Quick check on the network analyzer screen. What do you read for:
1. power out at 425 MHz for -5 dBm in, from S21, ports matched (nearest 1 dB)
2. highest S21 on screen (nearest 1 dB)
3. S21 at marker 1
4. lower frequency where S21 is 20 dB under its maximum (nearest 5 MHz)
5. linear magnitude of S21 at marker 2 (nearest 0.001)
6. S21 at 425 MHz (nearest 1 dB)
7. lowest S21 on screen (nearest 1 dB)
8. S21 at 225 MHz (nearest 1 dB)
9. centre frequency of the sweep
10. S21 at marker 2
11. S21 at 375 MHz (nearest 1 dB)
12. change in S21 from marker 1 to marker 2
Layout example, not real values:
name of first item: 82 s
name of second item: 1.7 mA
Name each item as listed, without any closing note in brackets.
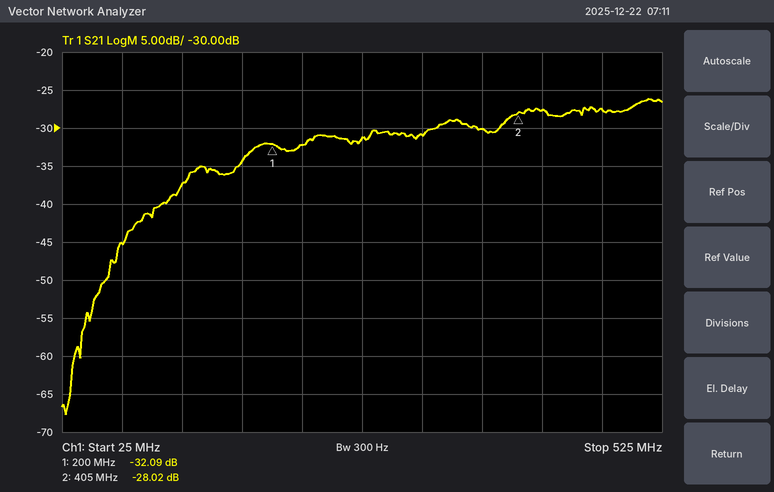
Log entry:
power out at 425 MHz for -5 dBm in, from S21, ports matched: -33 dBm
highest S21 on screen: -26 dB
S21 at marker 1: -32.09 dB
lower frequency where S21 is 20 dB under its maximum: 70 MHz
linear magnitude of S21 at marker 2: 0.040
S21 at 425 MHz: -28 dB
lowest S21 on screen: -68 dB
S21 at 225 MHz: -32 dB
centre frequency of the sweep: 275 MHz
S21 at marker 2: -28.02 dB
S21 at 375 MHz: -30 dB
change in S21 from marker 1 to marker 2: 4.07 dB
